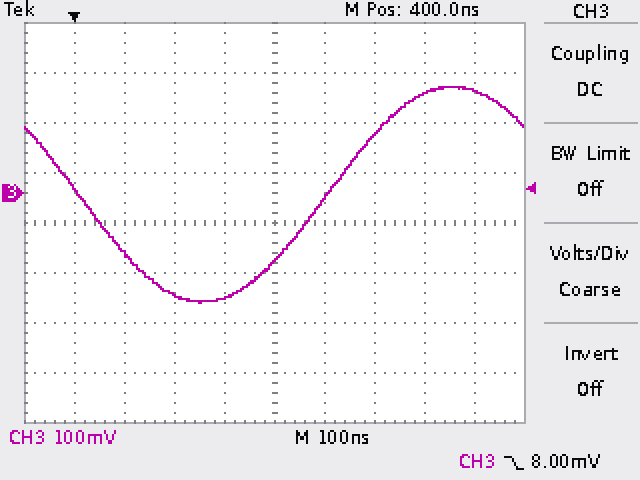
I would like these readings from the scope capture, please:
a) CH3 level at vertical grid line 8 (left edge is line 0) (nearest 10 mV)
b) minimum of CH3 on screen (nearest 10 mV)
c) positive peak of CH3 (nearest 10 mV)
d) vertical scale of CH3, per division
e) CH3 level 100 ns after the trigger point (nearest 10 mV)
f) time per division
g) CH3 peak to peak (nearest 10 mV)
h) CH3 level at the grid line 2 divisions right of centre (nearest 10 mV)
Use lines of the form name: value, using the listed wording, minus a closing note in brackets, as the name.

CH3 level at vertical grid line 8 (left edge is line 0): 200 mV
minimum of CH3 on screen: -220 mV
positive peak of CH3: 210 mV
vertical scale of CH3, per division: 100 mV
CH3 level 100 ns after the trigger point: -120 mV
time per division: 100 ns
CH3 peak to peak: 430 mV
CH3 level at the grid line 2 divisions right of centre: 120 mV
